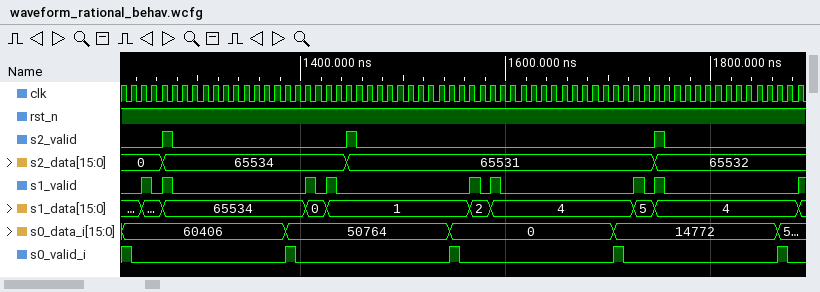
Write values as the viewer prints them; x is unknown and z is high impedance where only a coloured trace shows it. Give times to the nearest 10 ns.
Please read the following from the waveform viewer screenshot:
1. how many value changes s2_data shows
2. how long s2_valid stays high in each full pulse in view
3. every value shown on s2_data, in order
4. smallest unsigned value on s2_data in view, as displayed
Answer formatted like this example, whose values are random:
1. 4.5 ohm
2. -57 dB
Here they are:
1. 3
2. 10 ns, 10 ns, 10 ns
3. 0, 65534, 65531, 65532
4. 0
